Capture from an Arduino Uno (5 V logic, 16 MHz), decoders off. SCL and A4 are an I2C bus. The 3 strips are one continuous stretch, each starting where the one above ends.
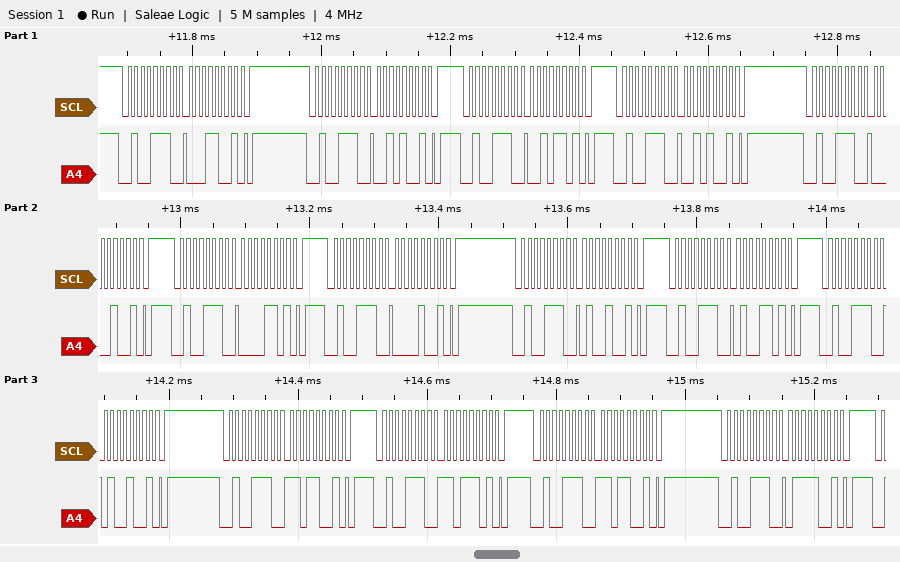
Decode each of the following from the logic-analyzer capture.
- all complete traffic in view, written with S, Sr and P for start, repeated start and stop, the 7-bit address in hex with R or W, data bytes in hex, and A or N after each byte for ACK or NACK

S 27W A 19 A P S 27W A 29 A P S 27W A 2D A P S 27W A 29 A P S 27W A 09 A P S 27W A 0D A P S 27W A 09 A P S 27W A 49 A P S 27W A 4D A P S 27W A 49 A P S 27W A D9 A P S 27W A DD A P S 27W A D9 A P S 27W A 79 A P
